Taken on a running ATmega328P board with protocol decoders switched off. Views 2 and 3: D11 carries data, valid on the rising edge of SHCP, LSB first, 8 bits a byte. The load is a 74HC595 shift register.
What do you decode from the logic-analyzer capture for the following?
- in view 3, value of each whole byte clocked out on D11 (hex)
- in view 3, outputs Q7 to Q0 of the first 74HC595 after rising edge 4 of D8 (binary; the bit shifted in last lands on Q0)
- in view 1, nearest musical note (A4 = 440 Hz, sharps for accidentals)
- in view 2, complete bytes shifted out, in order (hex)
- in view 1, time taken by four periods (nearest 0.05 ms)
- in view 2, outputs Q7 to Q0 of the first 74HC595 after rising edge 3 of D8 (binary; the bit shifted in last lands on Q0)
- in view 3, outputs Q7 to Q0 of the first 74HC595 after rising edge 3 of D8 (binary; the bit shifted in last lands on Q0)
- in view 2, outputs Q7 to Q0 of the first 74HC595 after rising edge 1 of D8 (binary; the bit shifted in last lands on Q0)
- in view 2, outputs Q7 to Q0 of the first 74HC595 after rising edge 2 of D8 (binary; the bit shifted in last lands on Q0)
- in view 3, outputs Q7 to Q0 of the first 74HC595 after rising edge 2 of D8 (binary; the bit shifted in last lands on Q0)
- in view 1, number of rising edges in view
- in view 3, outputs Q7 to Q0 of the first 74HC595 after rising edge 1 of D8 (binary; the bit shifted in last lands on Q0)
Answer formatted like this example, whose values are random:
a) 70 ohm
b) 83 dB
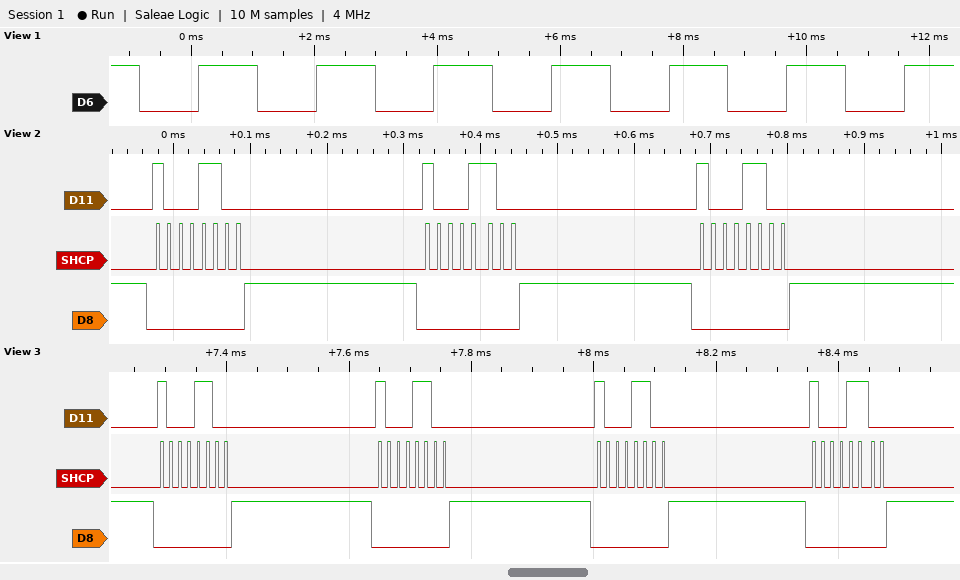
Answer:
a) 31 31 31 31
b) 10001100
c) C5
d) 31 31 31
e) 7.65 ms
f) 10001100
g) 10001100
h) 10001100
i) 10001100
j) 10001100
k) 7
l) 10001100
